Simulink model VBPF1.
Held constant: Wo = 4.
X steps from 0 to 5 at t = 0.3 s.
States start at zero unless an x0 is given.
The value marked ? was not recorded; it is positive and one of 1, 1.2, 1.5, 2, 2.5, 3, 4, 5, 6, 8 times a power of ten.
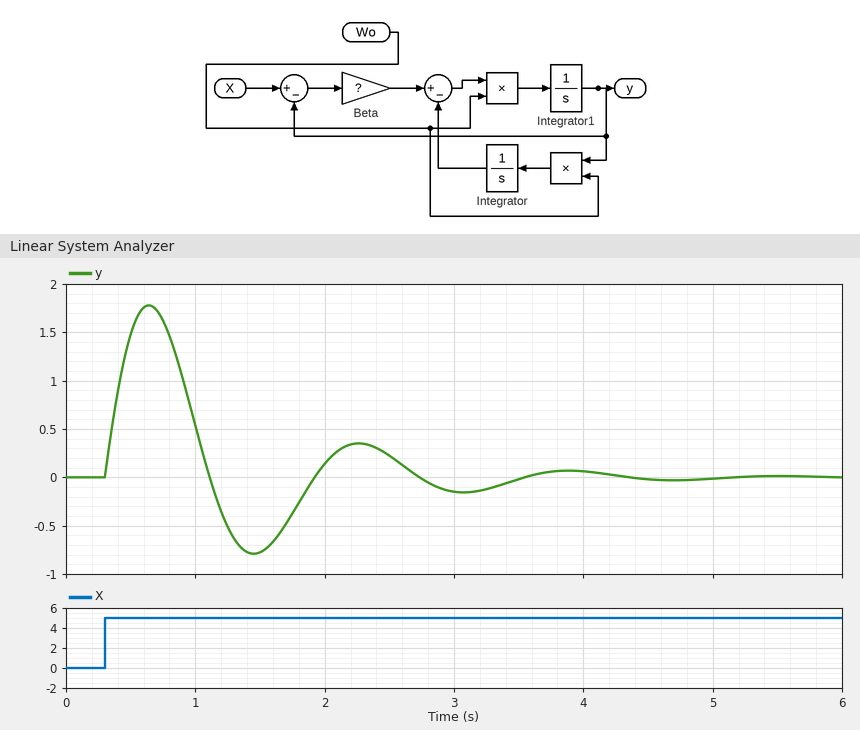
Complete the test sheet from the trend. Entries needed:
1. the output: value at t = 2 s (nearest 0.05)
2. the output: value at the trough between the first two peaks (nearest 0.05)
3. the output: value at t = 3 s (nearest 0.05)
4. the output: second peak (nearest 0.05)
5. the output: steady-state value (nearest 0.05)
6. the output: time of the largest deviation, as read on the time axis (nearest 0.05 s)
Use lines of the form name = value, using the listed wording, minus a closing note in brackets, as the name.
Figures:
the output: value at t = 2 s = 0.15
the output: value at the trough between the first two peaks = -0.80
the output: value at t = 3 s = -0.15
the output: second peak = 0.35
the output: steady-state value = 0.00
the output: time of the largest deviation, as read on the time axis = 0.65 s
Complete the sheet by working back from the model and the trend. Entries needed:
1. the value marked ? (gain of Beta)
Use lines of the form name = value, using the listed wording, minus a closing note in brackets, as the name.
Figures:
the value marked ? = 0.5
